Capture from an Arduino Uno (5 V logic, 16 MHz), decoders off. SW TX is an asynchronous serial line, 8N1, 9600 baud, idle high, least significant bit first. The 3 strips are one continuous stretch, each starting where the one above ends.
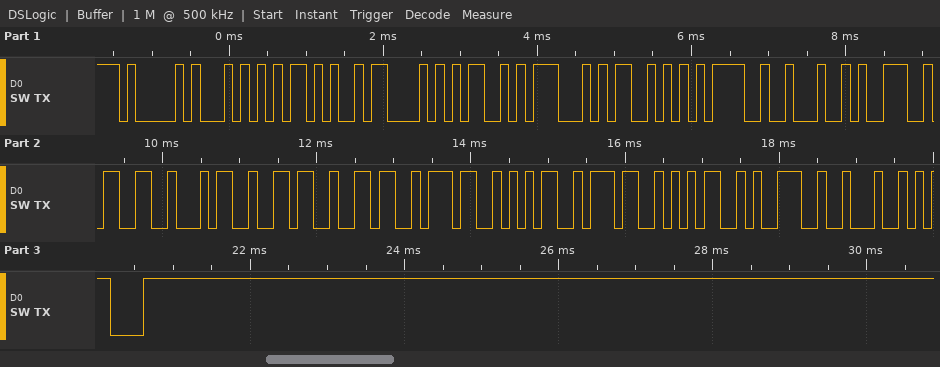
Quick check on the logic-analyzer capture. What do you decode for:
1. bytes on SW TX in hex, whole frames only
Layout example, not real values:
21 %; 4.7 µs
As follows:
0x41 0x54 0x2B 0x43 0x4D 0x47 0x53 0x3D 0x22 0x39 0x33 0x34 0x36 0x36 0x37 0x35 0x37 0x35 0x39 0x22 0x0D
